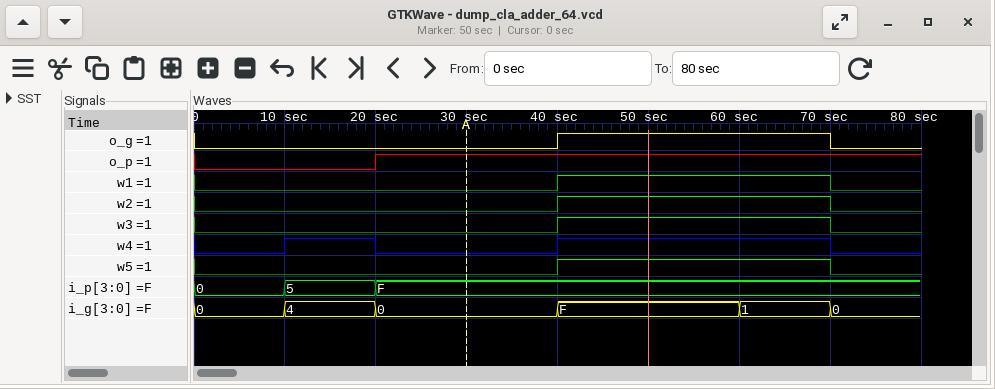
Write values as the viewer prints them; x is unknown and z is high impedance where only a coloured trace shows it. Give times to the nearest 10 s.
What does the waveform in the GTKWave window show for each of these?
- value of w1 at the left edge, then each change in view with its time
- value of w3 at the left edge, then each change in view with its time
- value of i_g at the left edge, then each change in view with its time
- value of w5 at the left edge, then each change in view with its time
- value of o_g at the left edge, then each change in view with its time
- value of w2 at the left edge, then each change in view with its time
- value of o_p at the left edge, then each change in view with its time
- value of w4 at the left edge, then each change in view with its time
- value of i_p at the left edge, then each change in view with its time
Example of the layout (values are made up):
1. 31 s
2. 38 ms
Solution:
1. 0, 1 at 40 s, 0 at 70 s
2. 0, 1 at 40 s, 0 at 70 s
3. 0, 4 at 10 s, 0 at 20 s, F at 40 s, 1 at 60 s, 0 at 70 s
4. 0, 1 at 40 s, 0 at 70 s
5. 0, 1 at 40 s, 0 at 70 s
6. 0, 1 at 40 s, 0 at 70 s
7. 0, 1 at 20 s
8. 0, 1 at 10 s, 0 at 20 s, 1 at 40 s, 0 at 70 s
9. 0, 5 at 10 s, F at 20 s
